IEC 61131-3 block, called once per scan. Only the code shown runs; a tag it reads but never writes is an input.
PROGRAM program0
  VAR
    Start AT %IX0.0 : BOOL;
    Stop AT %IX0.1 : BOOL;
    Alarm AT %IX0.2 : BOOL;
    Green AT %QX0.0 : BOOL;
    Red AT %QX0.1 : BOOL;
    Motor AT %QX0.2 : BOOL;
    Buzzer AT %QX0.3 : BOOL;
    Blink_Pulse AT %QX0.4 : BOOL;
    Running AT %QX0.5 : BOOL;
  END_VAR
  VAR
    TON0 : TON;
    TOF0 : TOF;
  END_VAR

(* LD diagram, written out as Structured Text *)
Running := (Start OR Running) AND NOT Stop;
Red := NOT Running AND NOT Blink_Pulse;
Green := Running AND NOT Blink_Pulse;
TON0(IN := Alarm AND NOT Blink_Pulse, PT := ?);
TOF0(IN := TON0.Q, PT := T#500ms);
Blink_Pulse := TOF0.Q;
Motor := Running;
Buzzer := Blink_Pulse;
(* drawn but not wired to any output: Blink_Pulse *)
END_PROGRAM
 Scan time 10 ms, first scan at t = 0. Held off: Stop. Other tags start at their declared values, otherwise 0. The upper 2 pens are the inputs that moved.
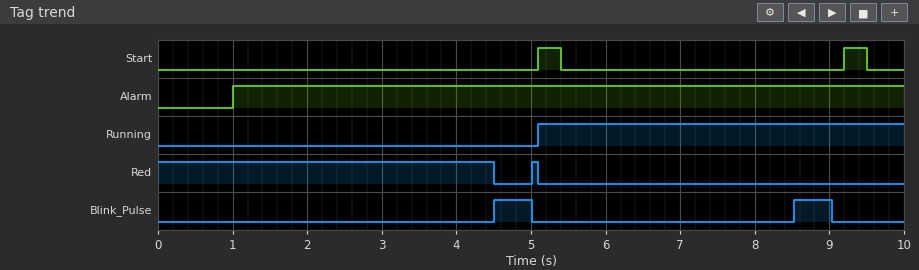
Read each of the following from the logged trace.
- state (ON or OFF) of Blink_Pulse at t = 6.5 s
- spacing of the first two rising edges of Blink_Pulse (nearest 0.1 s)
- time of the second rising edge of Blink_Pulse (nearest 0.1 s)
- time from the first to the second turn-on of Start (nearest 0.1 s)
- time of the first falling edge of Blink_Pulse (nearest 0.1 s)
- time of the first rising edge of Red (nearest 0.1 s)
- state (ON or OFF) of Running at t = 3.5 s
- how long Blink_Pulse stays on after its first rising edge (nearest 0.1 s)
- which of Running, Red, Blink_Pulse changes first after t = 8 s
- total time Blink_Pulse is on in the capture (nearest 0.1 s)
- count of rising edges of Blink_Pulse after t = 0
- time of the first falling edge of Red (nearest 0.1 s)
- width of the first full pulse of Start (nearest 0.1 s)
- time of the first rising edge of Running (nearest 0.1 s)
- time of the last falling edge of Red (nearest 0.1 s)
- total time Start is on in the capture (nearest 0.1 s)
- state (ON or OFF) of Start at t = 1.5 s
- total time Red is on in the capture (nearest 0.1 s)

OFF
4.0 s
8.5 s
4.1 s
5.0 s
5.0 s
OFF
0.5 s
Blink_Pulse
1.0 s
2
4.5 s
0.3 s
5.1 s
5.1 s
0.6 s
OFF
4.6 s
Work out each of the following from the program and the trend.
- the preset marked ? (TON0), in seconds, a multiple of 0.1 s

3.5 s
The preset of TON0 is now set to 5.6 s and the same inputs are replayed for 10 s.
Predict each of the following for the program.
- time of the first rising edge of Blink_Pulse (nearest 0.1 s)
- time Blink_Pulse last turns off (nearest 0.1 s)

6.6 s
7.1 s
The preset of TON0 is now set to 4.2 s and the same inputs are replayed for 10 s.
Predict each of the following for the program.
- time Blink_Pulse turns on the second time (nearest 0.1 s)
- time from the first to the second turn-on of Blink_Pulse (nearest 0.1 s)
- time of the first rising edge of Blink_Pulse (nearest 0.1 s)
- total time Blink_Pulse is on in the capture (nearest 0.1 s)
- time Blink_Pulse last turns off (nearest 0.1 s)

9.9 s
4.7 s
5.2 s
0.6 s
5.7 s
